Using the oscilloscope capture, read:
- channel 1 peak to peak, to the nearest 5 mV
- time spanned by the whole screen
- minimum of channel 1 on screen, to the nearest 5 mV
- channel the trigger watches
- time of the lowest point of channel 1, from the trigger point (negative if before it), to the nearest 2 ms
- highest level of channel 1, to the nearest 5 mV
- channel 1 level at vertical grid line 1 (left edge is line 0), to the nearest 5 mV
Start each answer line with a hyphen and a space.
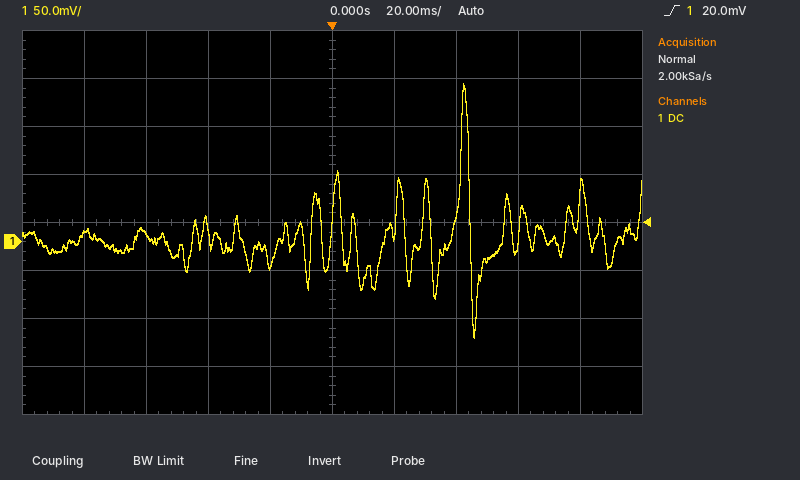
- 265 mV
- 200 ms
- -100 mV
- channel 1
- +46 ms
- 165 mV
- 10 mV
